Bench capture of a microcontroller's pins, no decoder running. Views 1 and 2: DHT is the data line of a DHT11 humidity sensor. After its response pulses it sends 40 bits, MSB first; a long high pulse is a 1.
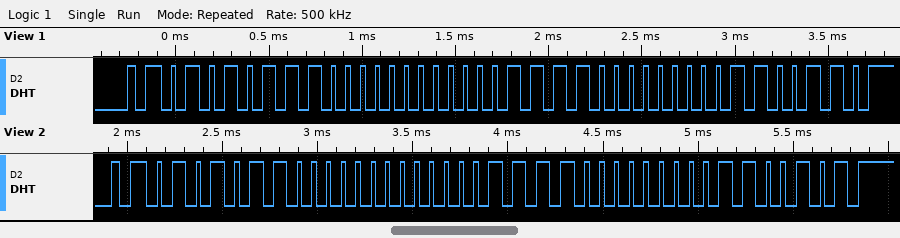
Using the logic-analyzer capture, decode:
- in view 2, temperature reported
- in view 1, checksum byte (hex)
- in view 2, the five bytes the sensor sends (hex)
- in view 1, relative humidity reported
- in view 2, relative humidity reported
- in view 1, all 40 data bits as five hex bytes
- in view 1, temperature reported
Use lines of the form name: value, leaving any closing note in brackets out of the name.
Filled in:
in view 2, temperature reported: 15.0 °C
in view 1, checksum byte: 0x66
in view 2, the five bytes the sensor sends: 56 00 0F 00 65
in view 1, relative humidity reported: 87 %
in view 2, relative humidity reported: 86 %
in view 1, all 40 data bits as five hex bytes: 57 00 0F 00 66
in view 1, temperature reported: 15.0 °C
